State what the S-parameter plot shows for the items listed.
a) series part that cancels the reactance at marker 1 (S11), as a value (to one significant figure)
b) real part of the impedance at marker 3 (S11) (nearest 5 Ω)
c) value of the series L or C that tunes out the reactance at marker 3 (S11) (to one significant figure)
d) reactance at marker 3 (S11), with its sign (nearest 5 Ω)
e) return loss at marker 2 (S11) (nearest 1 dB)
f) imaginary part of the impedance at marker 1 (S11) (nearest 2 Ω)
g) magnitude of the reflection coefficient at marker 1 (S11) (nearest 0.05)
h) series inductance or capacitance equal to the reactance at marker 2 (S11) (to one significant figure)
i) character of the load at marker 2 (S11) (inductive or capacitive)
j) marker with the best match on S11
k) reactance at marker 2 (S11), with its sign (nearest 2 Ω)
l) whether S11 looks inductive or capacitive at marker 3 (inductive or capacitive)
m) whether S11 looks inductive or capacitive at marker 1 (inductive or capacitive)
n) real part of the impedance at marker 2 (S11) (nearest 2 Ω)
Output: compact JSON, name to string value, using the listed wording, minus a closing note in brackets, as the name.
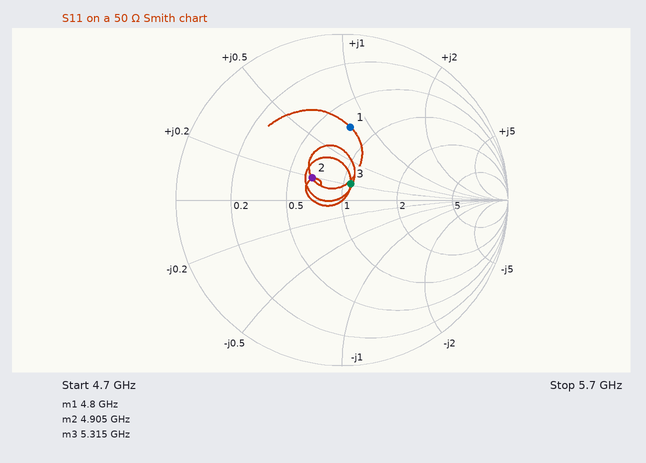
{"series part that cancels the reactance at marker 1 (S11), as a value": "800 fF", "real part of the impedance at marker 3 (S11)": "55 Ω", "value of the series L or C that tunes out the reactance at marker 3 (S11)": "3 pF", "reactance at marker 3 (S11), with its sign": "+10 Ω", "return loss at marker 2 (S11)": "13 dB", "imaginary part of the impedance at marker 1 (S11)": "+40 Ω", "magnitude of the reflection coefficient at marker 1 (S11)": "0.45", "series inductance or capacitance equal to the reactance at marker 2 (S11)": "300 pH", "character of the load at marker 2 (S11)": "inductive", "marker with the best match on S11": "marker 3", "reactance at marker 2 (S11), with its sign": "+10 Ω", "whether S11 looks inductive or capacitive at marker 3": "inductive", "whether S11 looks inductive or capacitive at marker 1": "inductive", "real part of the impedance at marker 2 (S11)": "34 Ω"}
